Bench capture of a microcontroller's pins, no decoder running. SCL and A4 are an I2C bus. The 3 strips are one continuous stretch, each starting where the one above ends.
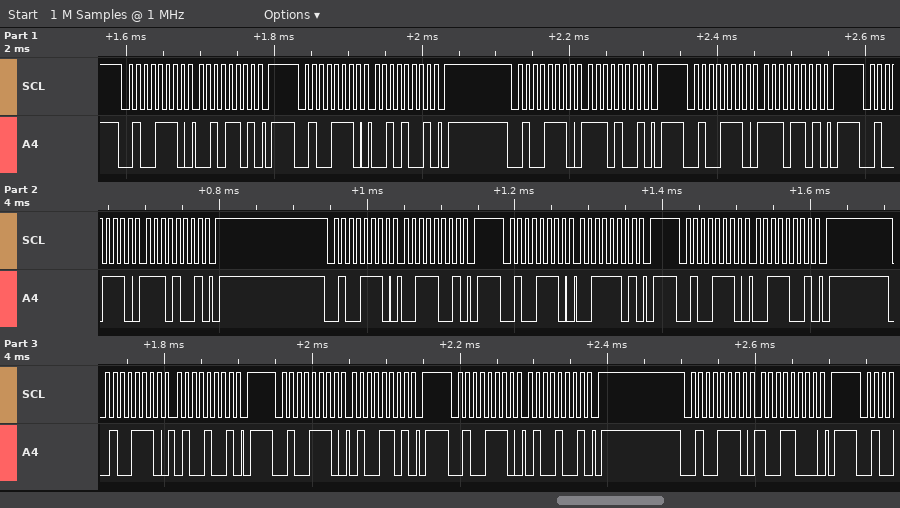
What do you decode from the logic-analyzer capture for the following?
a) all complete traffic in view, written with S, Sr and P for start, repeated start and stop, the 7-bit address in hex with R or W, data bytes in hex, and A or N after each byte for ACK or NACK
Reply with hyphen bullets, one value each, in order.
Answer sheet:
- S 27W A 2D A P S 27W A 29 A P S 27W A E9 A P S 27W A ED A P S 27W A E9 A P S 27W A 39 A P S 27W A 3D A P S 27W A 39 A P S 27W A 49 A P S 27W A 4D A P S 27W A 49 A P S 27W A 98 A P
